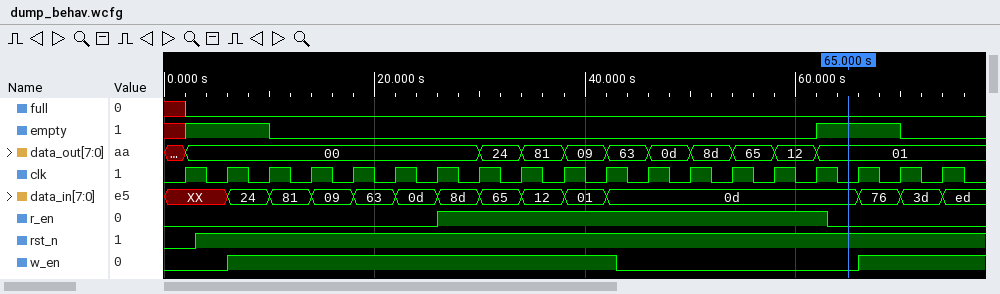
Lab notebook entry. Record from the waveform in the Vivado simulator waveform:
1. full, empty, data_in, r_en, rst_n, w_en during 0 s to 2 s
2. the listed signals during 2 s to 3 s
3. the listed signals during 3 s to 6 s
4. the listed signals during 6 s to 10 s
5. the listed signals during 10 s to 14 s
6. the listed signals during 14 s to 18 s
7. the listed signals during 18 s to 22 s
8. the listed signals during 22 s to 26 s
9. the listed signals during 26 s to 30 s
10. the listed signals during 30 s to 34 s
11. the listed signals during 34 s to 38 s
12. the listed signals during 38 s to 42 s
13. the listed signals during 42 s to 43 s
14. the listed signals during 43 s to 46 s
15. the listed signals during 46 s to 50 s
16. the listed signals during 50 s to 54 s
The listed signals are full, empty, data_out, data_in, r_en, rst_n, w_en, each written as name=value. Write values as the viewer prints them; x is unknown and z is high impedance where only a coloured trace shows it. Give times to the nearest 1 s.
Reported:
full=x, empty=x, data_in=XX, r_en=0, rst_n=0, w_en=0
full=0, empty=1, data_out=00, data_in=XX, r_en=0, rst_n=0, w_en=0
full=0, empty=1, data_out=00, data_in=XX, r_en=0, rst_n=1, w_en=0
full=0, empty=1, data_out=00, data_in=24, r_en=0, rst_n=1, w_en=1
full=0, empty=0, data_out=00, data_in=81, r_en=0, rst_n=1, w_en=1
full=0, empty=0, data_out=00, data_in=09, r_en=0, rst_n=1, w_en=1
full=0, empty=0, data_out=00, data_in=63, r_en=0, rst_n=1, w_en=1
full=0, empty=0, data_out=00, data_in=0d, r_en=0, rst_n=1, w_en=1
full=0, empty=0, data_out=00, data_in=8d, r_en=1, rst_n=1, w_en=1
full=0, empty=0, data_out=24, data_in=65, r_en=1, rst_n=1, w_en=1
full=0, empty=0, data_out=81, data_in=12, r_en=1, rst_n=1, w_en=1
full=0, empty=0, data_out=09, data_in=01, r_en=1, rst_n=1, w_en=1
full=0, empty=0, data_out=63, data_in=0d, r_en=1, rst_n=1, w_en=1
full=0, empty=0, data_out=63, data_in=0d, r_en=1, rst_n=1, w_en=0
full=0, empty=0, data_out=0d, data_in=0d, r_en=1, rst_n=1, w_en=0
full=0, empty=0, data_out=8d, data_in=0d, r_en=1, rst_n=1, w_en=0
